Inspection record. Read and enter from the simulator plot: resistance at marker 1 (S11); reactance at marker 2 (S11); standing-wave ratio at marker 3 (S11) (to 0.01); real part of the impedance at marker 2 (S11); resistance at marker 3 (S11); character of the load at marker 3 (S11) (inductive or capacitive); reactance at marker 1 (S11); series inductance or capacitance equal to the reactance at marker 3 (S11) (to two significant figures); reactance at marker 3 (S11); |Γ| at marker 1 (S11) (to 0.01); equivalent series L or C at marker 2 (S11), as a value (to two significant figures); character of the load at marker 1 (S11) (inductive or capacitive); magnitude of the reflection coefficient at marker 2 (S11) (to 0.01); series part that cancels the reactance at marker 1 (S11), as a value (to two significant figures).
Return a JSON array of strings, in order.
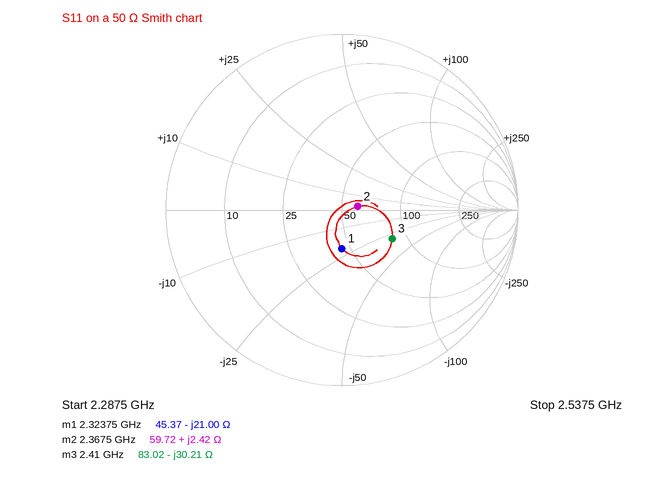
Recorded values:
["45.37 Ω", "+2.42 Ω", "1.98", "59.72 Ω", "83.02 Ω", "capacitive", "-21.00 Ω", "2.2 pF", "-30.21 Ω", "0.22", "160 pH", "capacitive", "0.09", "1.4 nH"]
